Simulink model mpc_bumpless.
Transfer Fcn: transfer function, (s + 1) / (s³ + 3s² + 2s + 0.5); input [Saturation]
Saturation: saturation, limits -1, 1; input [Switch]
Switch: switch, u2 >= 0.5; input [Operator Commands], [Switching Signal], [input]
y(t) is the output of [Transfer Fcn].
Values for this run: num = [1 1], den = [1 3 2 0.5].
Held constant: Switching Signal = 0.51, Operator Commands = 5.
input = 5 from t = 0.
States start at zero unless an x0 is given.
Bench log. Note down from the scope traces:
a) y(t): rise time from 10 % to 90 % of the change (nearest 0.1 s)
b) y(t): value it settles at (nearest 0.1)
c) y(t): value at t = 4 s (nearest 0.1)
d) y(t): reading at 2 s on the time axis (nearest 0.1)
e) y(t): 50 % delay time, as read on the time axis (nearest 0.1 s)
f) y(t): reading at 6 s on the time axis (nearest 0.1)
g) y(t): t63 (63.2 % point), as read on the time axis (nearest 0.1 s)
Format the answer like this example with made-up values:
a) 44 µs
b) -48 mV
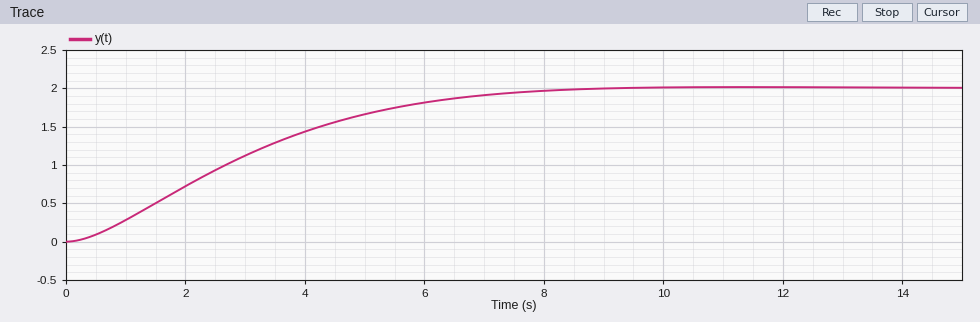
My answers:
a) 5.1 s
b) 2.0
c) 1.4
d) 0.7
e) 2.7 s
f) 1.8
g) 3.4 s
